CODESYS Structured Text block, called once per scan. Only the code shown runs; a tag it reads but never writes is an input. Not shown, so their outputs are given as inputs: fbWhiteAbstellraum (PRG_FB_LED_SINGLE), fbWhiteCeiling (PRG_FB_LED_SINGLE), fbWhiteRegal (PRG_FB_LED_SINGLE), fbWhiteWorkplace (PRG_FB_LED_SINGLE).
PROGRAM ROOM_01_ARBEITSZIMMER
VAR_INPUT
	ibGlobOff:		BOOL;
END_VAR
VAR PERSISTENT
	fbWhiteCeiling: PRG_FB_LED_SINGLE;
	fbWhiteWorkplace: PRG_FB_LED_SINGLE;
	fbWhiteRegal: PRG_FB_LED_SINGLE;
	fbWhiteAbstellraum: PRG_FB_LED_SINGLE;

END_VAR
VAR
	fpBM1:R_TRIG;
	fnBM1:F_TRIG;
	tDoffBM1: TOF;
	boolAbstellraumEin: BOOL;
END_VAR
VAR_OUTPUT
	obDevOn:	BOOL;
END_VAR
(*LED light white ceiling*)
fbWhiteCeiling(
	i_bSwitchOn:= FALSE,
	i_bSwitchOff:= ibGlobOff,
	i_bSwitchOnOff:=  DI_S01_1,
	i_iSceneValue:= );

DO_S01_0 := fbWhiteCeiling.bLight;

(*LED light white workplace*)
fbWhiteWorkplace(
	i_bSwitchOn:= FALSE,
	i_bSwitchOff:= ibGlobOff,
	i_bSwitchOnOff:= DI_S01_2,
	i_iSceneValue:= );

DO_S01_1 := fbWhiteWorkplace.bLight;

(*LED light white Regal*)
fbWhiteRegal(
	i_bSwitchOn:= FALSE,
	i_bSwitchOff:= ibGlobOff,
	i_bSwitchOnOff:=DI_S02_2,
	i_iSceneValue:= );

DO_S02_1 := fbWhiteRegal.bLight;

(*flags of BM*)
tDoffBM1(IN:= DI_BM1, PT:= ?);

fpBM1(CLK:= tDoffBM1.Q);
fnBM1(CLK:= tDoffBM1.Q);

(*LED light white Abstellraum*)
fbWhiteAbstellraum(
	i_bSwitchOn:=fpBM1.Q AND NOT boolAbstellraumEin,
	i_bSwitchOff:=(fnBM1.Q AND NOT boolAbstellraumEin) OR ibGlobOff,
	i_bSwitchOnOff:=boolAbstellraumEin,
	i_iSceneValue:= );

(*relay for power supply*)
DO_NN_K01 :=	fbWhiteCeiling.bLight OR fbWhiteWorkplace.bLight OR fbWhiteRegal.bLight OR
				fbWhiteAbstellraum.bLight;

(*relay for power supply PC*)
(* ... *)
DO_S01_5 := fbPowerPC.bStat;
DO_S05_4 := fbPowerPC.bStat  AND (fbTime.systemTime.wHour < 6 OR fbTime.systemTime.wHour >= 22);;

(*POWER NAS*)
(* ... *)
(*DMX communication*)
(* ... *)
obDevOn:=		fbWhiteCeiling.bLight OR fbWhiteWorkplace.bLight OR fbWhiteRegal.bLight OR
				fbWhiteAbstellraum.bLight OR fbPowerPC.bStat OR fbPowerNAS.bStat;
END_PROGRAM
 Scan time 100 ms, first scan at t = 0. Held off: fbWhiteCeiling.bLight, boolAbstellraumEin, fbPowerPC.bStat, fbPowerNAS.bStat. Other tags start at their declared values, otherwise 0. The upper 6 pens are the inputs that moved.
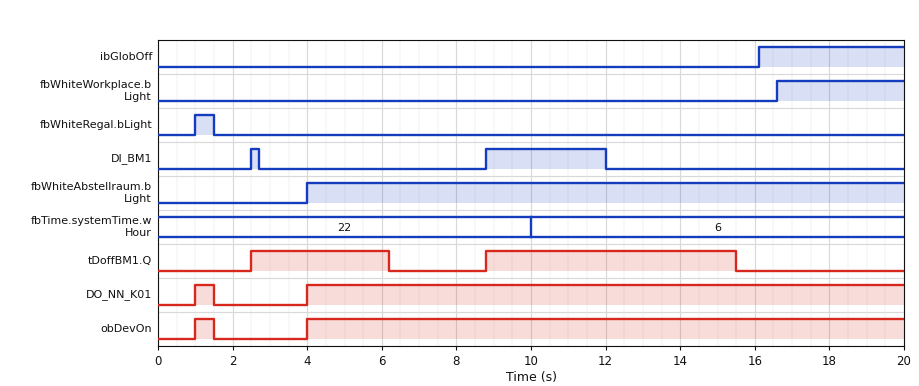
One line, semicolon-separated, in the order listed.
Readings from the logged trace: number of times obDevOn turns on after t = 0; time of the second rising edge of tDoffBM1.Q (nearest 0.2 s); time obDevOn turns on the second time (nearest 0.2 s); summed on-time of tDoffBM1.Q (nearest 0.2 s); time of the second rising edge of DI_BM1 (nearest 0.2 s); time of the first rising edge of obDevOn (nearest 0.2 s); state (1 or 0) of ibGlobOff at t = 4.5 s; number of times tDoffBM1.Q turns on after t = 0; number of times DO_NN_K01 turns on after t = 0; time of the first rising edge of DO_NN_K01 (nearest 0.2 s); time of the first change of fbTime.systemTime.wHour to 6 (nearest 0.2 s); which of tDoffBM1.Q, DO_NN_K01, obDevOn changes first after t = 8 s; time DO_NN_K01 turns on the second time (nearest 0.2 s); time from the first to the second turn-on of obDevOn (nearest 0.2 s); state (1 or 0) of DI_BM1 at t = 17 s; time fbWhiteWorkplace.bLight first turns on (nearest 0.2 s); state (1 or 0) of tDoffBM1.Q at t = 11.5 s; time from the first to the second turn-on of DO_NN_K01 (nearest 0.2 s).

2; 8.8 s; 4.0 s; 10.4 s; 8.8 s; 1.0 s; 0; 2; 2; 1.0 s; 10.0 s; tDoffBM1.Q; 4.0 s; 3.0 s; 0; 16.6 s; 1; 3.0 s
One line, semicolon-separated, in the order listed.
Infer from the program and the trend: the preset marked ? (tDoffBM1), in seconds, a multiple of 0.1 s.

3.5 s
